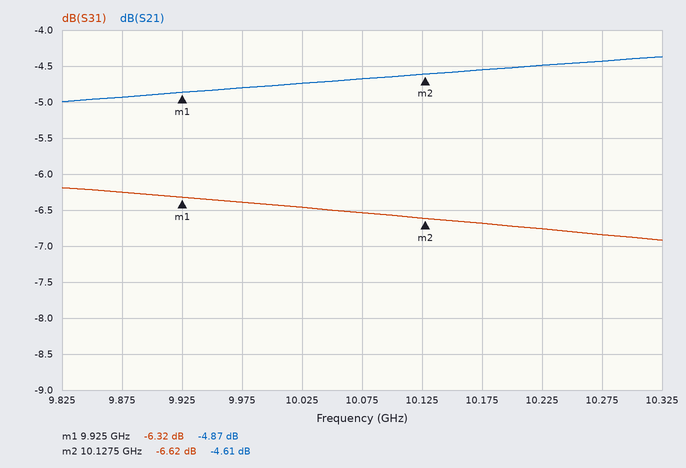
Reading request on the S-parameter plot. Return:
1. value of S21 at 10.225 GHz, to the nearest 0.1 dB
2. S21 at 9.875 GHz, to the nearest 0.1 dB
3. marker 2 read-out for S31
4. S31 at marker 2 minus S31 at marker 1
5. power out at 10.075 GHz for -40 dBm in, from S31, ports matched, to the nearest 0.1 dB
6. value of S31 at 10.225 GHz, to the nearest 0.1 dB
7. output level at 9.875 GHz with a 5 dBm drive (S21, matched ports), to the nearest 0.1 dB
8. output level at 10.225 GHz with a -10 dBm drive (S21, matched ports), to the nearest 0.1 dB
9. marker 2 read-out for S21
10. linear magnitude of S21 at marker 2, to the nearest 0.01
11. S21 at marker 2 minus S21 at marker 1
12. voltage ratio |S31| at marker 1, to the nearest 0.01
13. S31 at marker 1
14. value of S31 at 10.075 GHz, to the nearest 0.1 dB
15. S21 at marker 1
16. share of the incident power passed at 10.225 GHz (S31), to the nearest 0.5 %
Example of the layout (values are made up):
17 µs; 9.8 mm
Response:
-4.5 dB; -4.9 dB; -6.62 dB; -0.30 dB; -46.5 dBm; -6.8 dB; 0.1 dBm; -14.5 dBm; -4.61 dB; 0.59; 0.26 dB; 0.48; -6.32 dB; -6.5 dB; -4.87 dB; 21.0 %
